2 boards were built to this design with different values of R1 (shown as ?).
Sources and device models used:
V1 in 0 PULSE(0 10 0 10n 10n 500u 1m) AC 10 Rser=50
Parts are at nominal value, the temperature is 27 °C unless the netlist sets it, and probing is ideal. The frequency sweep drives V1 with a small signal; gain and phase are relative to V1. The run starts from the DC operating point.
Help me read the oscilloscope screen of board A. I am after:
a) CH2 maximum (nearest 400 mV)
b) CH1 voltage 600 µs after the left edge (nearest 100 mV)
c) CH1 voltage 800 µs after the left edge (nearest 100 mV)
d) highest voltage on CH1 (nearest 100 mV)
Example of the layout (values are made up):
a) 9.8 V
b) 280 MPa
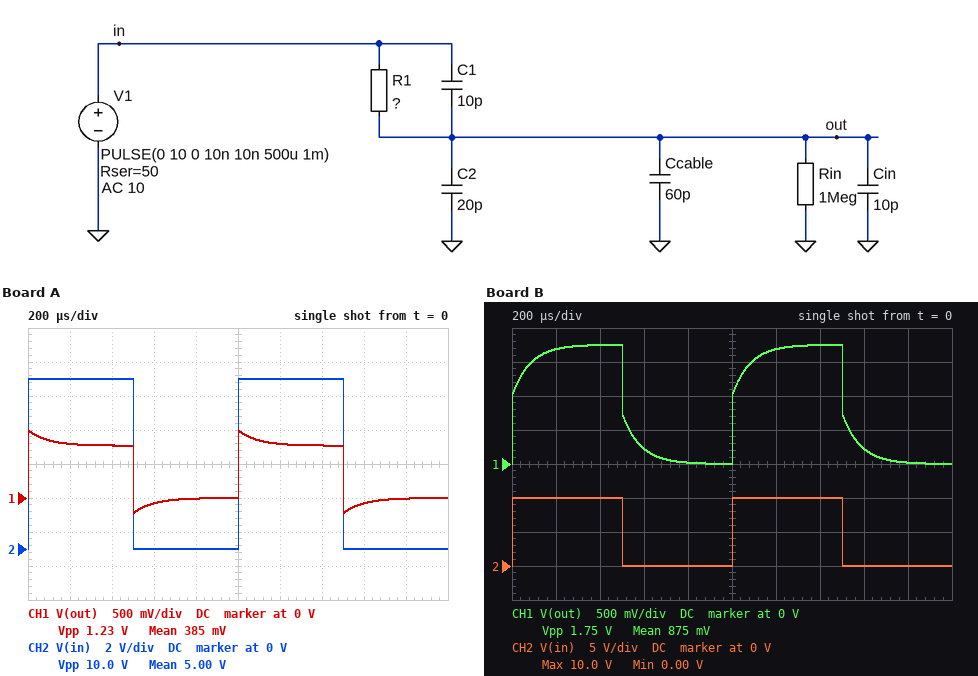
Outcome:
a) 10.0 V
b) -100 mV
c) 0 V
d) 1.0 V
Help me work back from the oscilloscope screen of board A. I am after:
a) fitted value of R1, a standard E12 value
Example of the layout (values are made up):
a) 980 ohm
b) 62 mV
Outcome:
a) 12 MΩ
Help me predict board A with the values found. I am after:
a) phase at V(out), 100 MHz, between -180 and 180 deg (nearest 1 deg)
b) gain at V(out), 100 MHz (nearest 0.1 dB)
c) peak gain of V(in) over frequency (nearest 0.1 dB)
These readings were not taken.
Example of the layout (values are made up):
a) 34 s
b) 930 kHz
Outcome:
a) -16 deg
b) -20.3 dB
c) 0 dB
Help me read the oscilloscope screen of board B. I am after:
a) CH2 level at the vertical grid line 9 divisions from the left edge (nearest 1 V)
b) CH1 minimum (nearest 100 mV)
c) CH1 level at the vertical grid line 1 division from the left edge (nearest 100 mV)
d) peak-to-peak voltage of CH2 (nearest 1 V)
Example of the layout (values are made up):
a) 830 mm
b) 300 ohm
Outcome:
a) 0 V
b) 0 V
c) 1.7 V
d) 10 V
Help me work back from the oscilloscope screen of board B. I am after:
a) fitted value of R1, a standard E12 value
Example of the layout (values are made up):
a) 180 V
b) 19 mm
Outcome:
a) 4.7 MΩ
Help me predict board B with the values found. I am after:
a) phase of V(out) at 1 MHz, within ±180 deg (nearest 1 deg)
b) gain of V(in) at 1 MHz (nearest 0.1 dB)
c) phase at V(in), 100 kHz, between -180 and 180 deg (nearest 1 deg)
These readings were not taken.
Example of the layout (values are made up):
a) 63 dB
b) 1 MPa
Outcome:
a) 0 deg
b) 0 dB
c) 0 deg
